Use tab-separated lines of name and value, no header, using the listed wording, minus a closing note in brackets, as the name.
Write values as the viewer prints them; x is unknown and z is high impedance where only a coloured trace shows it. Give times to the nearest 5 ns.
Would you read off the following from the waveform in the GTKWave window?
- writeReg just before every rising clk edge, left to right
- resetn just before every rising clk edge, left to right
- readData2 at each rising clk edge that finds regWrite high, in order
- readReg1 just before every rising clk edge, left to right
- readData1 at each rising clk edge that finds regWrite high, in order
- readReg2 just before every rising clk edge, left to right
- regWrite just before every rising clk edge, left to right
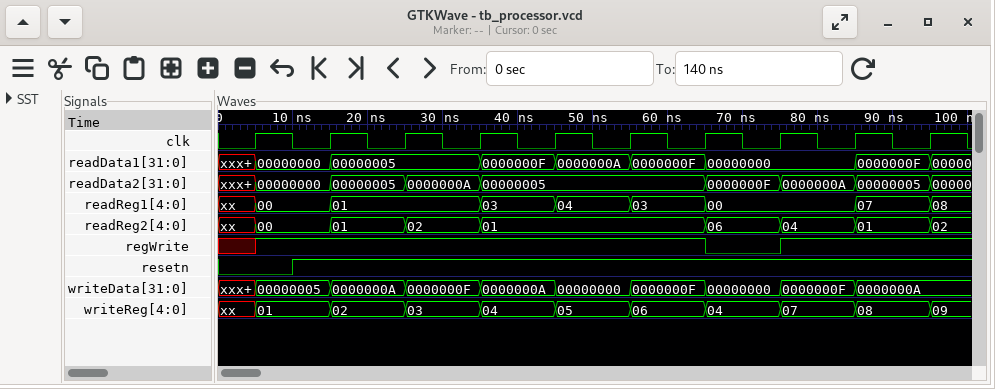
writeReg just before every rising clk edge, left to right	xx, 01, 02, 03, 04, 05, 06, 04, 07, 08
resetn just before every rising clk edge, left to right	0 1 1 1 1 1 1 1 1 1
readData2 at each rising clk edge that finds regWrite high, in order	00000000, 00000005, 0000000A, 00000005, 00000005, 00000005, 0000000A, 00000005
readReg1 just before every rising clk edge, left to right	xx, 00, 01, 01, 03, 04, 03, 00, 00, 07
readData1 at each rising clk edge that finds regWrite high, in order	00000000, 00000005, 00000005, 0000000F, 0000000A, 0000000F, 00000000, 0000000F
readReg2 just before every rising clk edge, left to right	xx, 00, 01, 02, 01, 01, 01, 06, 04, 01
regWrite just before every rising clk edge, left to right	x 1 1 1 1 1 1 0 1 1
